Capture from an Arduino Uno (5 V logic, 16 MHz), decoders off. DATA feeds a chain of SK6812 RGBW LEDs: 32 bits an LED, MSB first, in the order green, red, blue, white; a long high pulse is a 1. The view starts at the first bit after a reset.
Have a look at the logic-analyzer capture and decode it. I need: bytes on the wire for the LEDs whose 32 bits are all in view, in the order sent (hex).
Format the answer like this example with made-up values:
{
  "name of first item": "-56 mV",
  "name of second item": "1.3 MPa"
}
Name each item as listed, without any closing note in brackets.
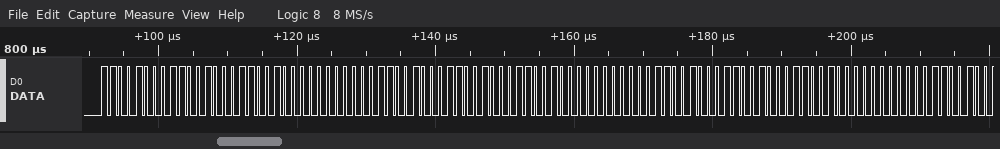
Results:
{
  "bytes on the wire for the LEDs whose 32 bits are all in view, in the order sent": "C8 C8 C8 00 C8 C8 C8 00 C8 C8 C8 00"
}
